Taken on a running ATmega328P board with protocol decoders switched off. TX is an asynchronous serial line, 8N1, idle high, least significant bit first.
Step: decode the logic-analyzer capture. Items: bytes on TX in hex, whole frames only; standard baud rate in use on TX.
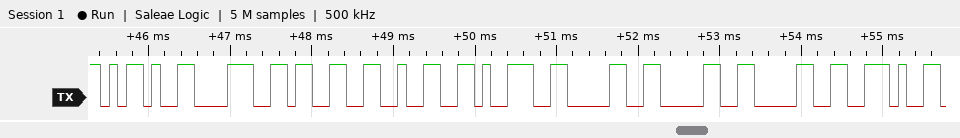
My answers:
0x2D 0x38 0x33 0x32 0x39 0x30 0x30 0x30 0x2E
9600 baud
